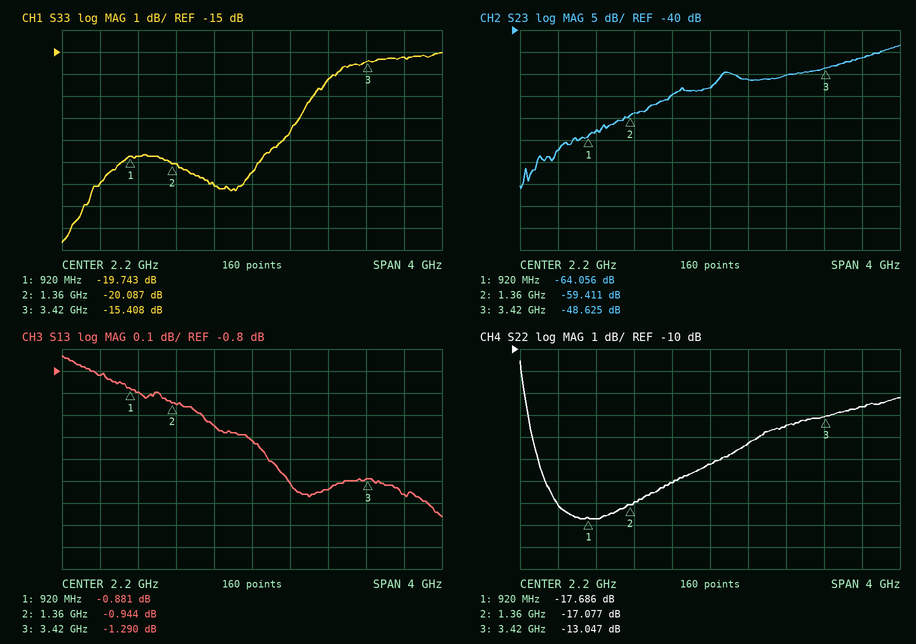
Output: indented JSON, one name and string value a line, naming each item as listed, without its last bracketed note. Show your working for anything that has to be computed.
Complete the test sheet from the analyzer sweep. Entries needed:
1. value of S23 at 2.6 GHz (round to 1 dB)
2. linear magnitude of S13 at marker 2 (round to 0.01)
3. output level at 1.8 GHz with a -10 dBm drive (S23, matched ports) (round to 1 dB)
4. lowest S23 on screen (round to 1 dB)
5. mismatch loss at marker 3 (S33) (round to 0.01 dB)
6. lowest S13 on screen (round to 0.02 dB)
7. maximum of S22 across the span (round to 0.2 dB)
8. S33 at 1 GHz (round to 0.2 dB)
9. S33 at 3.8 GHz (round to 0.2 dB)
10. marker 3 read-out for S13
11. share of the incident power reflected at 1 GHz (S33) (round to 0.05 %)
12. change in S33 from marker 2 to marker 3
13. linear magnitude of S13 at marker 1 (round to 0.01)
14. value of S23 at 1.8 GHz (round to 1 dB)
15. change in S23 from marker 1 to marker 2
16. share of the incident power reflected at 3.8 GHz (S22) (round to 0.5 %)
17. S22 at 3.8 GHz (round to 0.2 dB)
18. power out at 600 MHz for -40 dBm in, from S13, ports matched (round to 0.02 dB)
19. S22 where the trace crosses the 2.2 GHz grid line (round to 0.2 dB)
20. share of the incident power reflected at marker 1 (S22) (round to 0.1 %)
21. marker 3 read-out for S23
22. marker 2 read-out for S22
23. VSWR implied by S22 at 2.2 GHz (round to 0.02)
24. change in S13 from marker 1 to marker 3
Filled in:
{
  "value of S23 at 2.6 GHz": "-51 dB",
  "linear magnitude of S13 at marker 2": "10^(-0.944/20) ≈ 0.90",
  "output level at 1.8 GHz with a -10 dBm drive (S23, matched ports)": "-10 dBm + (-55 dB) = -65 dBm",
  "lowest S23 on screen": "-76 dB",
  "mismatch loss at marker 3 (S33)": "−10 log10(1 − 10^(-15.408/10)) ≈ 0.13 dB",
  "lowest S13 on screen": "-1.46 dB",
  "maximum of S22 across the span": "-10.6 dB",
  "S33 at 1 GHz": "-19.8 dB",
  "S33 at 3.8 GHz": "-15.2 dB",
  "marker 3 read-out for S13": "-1.290 dB",
  "share of the incident power reflected at 1 GHz (S33)": "10^(-19.8/10) ≈ 1.05 %",
  "change in S33 from marker 2 to marker 3": "-15.408 − (-20.087) = 4.679 dB",
  "linear magnitude of S13 at marker 1": "10^(-0.881/20) ≈ 0.90",
  "value of S23 at 1.8 GHz": "-55 dB",
  "change in S23 from marker 1 to marker 2": "-59.411 − (-64.056) = 4.645 dB",
  "share of the incident power reflected at 3.8 GHz (S22)": "10^(-12.6/10) ≈ 5.5 %",
  "S22 at 3.8 GHz": "-12.6 dB",
  "power out at 600 MHz for -40 dBm in, from S13, ports matched": "-40 dBm + (-0.82 dB) = -40.82 dBm",
  "S22 where the trace crosses the 2.2 GHz grid line": "-15.2 dB",
  "share of the incident power reflected at marker 1 (S22)": "10^(-17.686/10) ≈ 1.7 %",
  "marker 3 read-out for S23": "-48.625 dB",
  "marker 2 read-out for S22": "-17.077 dB",
  "VSWR implied by S22 at 2.2 GHz": "|Γ| = 10^(-15.2/20) = 0.1738; VSWR = (1 + 0.1738)/(1 − 0.1738) ≈ 1.42",
  "change in S13 from marker 1 to marker 3": "-1.29 − (-0.881) = -0.409 dB"
}
